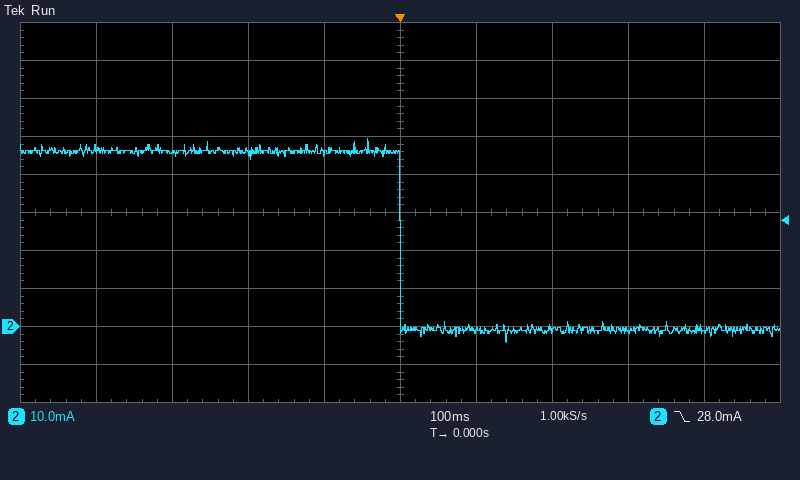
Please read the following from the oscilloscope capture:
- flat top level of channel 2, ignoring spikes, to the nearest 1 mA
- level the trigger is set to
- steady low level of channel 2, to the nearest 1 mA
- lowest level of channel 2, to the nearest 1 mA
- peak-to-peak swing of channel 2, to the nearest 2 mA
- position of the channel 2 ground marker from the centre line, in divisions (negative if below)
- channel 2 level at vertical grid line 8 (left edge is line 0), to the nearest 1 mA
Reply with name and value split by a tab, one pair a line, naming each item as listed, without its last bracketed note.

flat top level of channel 2, ignoring spikes, to the nearest 1 mA	46 mA
level the trigger is set to	28.0 mA
steady low level of channel 2, to the nearest 1 mA	-1 mA
lowest level of channel 2, to the nearest 1 mA	-4 mA
peak-to-peak swing of channel 2, to the nearest 2 mA	54 mA
position of the channel 2 ground marker from the centre line, in divisions	-3.0 div
channel 2 level at vertical grid line 8 (left edge is line 0), to the nearest 1 mA	-1 mA
